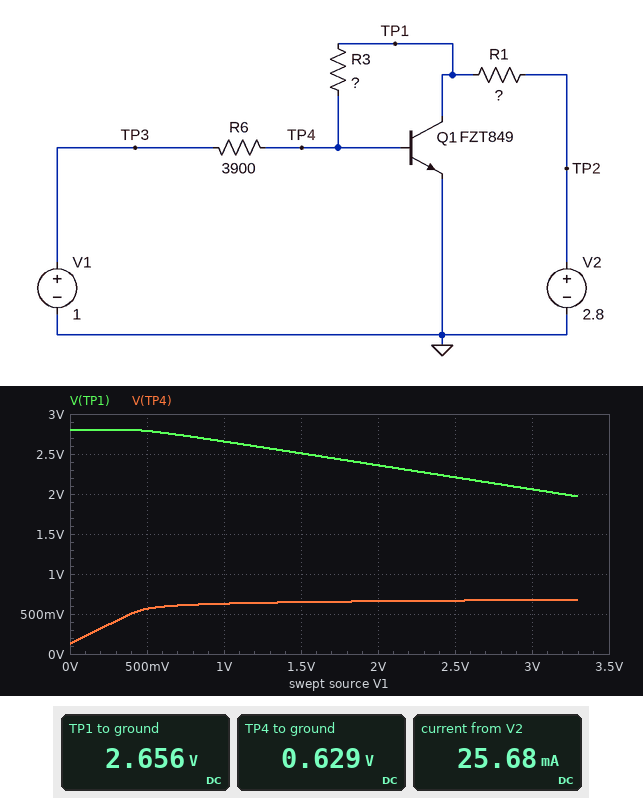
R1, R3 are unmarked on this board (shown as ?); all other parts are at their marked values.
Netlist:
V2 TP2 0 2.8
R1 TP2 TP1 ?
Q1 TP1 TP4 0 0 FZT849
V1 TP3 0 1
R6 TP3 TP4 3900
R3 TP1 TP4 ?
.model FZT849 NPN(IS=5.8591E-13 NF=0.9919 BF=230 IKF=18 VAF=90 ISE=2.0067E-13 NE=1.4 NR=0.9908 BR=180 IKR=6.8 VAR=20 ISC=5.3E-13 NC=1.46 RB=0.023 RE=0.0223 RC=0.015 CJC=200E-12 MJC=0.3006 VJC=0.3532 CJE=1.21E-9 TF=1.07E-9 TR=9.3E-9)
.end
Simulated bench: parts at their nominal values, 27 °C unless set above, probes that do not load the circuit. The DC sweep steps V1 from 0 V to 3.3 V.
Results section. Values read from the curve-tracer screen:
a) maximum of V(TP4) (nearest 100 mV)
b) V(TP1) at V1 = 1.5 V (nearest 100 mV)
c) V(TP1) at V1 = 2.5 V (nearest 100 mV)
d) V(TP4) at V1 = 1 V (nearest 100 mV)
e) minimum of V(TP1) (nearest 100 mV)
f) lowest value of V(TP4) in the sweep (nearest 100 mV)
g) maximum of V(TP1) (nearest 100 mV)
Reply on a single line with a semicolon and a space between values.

700 mV; 2.5 V; 2.2 V; 600 mV; 2.0 V; 100 mV; 2.8 V
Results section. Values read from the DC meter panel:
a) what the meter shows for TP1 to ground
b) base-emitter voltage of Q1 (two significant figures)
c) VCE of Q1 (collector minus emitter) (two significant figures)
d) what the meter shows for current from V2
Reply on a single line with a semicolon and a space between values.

2.656 V; 630 mV; 2.7 V; 25.68 mA
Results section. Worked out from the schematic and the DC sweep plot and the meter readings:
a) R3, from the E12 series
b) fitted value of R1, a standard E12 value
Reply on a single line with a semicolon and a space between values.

82 kΩ; 5.6 Ω
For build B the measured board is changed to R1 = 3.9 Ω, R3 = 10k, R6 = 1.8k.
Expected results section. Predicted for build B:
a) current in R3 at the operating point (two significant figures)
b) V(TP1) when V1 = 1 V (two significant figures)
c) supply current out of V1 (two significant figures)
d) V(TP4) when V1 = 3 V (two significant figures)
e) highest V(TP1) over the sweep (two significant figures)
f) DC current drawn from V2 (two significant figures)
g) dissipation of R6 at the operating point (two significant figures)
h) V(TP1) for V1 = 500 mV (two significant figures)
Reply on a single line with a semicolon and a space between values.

180 µA; 2.5 V; 190 µA; 700 mV; 2.8 V; 81 mA; 64 µW; 2.7 V
